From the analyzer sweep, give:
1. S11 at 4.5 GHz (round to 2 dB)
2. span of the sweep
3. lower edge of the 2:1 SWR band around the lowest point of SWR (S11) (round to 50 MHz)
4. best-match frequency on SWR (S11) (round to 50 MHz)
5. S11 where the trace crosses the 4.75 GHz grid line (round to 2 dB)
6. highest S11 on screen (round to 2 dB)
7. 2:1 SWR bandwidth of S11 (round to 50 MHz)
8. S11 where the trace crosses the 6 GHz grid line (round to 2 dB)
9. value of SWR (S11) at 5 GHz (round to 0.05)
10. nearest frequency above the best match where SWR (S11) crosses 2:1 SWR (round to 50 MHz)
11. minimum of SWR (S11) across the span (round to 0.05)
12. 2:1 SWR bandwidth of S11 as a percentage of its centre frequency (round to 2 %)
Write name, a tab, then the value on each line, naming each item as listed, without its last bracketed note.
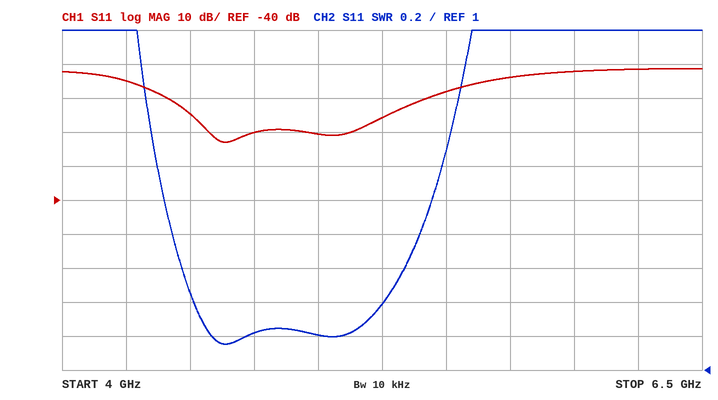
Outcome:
S11 at 4.5 GHz	-14 dB
span of the sweep	2.5 GHz
lower edge of the 2:1 SWR band around the lowest point of SWR (S11)	4.40 GHz
best-match frequency on SWR (S11)	4.65 GHz
S11 where the trace crosses the 4.75 GHz grid line	-20 dB
highest S11 on screen	-2 dB
2:1 SWR bandwidth of S11	1.05 GHz
S11 where the trace crosses the 6 GHz grid line	-2 dB
value of SWR (S11) at 5 GHz	1.20
nearest frequency above the best match where SWR (S11) crosses 2:1 SWR	5.45 GHz
minimum of SWR (S11) across the span	1.15
2:1 SWR bandwidth of S11 as a percentage of its centre frequency	22 %
